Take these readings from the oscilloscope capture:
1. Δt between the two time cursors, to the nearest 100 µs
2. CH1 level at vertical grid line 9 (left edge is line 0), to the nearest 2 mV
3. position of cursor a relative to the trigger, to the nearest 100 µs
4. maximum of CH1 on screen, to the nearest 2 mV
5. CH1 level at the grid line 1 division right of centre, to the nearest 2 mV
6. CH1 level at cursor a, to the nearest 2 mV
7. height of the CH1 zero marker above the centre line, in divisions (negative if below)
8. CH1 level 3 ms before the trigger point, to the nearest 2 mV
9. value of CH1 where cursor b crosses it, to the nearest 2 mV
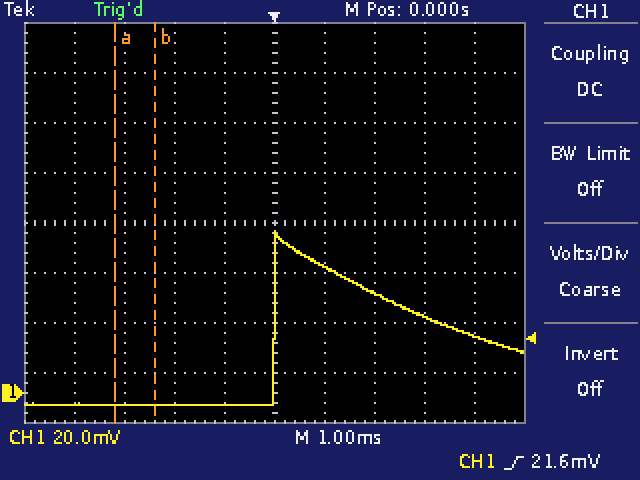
800 µs
22 mV
-3.2 ms
64 mV
50 mV
-4 mV
-3.4 div
-4 mV
-4 mV
